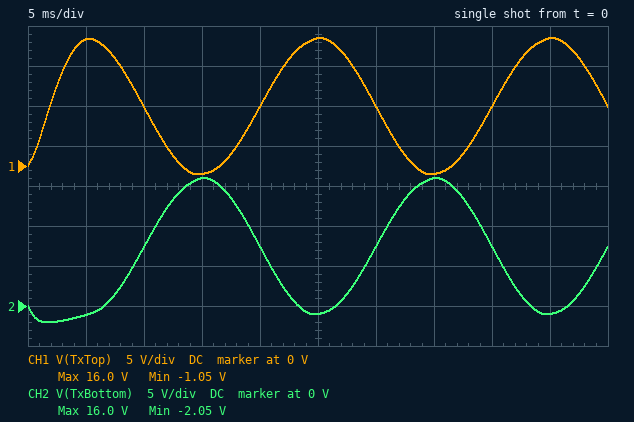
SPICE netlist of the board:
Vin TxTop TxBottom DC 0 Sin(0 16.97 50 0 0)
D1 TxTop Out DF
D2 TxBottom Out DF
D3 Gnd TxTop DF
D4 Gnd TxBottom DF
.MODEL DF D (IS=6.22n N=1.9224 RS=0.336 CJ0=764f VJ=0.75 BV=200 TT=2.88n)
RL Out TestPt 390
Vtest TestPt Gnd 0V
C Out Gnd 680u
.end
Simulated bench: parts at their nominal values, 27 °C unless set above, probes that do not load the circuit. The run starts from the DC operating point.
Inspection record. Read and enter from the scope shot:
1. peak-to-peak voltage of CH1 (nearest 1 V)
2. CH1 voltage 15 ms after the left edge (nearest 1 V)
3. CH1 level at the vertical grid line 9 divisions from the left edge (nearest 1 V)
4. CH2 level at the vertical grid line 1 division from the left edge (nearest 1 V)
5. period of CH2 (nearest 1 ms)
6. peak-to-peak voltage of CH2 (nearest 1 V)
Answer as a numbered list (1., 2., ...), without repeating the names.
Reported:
1. 17 V
2. -1 V
3. 16 V
4. -1 V
5. 20 ms
6. 18 V
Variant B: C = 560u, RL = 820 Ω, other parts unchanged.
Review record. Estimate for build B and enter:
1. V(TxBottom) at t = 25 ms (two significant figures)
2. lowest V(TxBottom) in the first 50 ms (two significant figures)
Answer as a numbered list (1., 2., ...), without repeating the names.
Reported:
1. -920 mV
2. -1.9 V
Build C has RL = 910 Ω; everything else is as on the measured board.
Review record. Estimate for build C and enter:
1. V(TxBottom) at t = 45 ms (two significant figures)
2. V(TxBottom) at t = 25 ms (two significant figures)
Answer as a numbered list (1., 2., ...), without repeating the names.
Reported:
1. -920 mV
2. -930 mV
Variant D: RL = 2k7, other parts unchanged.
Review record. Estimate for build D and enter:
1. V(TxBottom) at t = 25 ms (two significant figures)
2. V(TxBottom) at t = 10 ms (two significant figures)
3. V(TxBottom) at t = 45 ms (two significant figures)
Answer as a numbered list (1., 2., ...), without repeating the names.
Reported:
1. -880 mV
2. 7.5 V
3. -850 mV
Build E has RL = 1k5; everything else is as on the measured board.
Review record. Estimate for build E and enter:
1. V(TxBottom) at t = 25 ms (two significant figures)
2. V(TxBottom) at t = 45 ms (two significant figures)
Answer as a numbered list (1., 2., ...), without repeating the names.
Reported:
1. -900 mV
2. -880 mV
